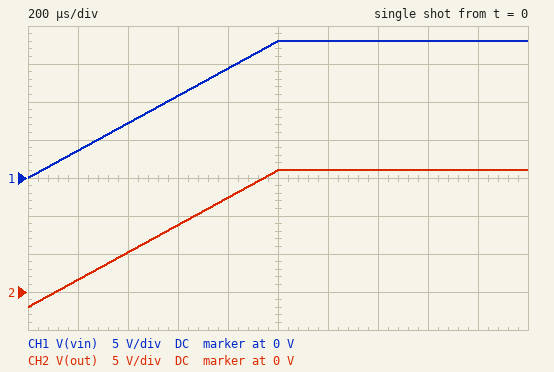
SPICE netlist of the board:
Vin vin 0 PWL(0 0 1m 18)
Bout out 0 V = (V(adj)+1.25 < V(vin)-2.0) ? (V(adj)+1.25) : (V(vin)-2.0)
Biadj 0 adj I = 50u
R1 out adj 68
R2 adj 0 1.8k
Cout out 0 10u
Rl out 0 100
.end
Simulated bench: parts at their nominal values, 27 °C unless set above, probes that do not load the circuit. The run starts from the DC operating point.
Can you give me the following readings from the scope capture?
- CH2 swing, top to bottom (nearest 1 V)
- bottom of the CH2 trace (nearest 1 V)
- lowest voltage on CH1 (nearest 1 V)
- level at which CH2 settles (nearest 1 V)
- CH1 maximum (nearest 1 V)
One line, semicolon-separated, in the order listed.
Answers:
18 V; -2 V; 0 V; 16 V; 18 V
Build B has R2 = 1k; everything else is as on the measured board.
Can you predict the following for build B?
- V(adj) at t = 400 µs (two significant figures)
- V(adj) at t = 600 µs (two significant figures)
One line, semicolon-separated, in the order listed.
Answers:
4.9 V; 8.2 V
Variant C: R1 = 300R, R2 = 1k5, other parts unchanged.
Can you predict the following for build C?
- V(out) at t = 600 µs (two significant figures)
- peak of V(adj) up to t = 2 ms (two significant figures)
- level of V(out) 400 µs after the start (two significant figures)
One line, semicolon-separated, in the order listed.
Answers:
7.6 V; 6.3 V; 5.2 V
